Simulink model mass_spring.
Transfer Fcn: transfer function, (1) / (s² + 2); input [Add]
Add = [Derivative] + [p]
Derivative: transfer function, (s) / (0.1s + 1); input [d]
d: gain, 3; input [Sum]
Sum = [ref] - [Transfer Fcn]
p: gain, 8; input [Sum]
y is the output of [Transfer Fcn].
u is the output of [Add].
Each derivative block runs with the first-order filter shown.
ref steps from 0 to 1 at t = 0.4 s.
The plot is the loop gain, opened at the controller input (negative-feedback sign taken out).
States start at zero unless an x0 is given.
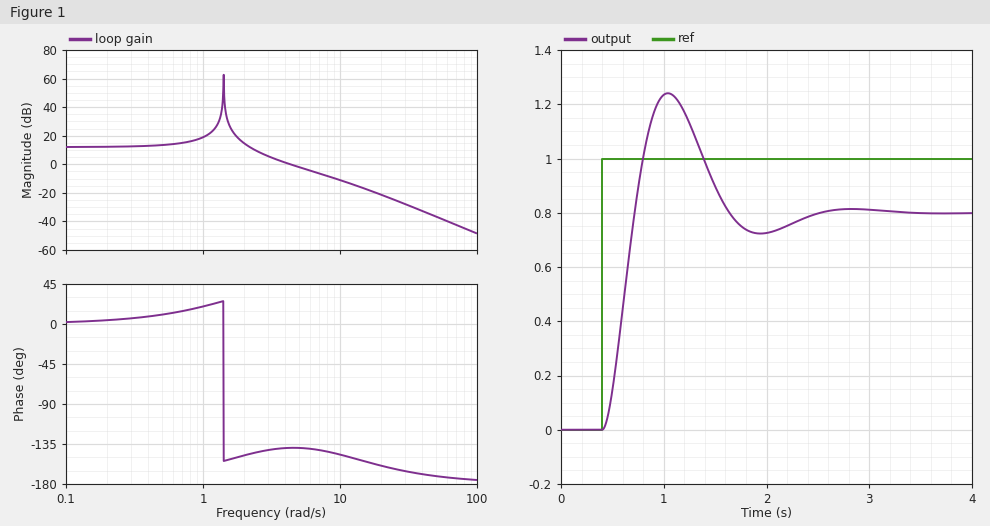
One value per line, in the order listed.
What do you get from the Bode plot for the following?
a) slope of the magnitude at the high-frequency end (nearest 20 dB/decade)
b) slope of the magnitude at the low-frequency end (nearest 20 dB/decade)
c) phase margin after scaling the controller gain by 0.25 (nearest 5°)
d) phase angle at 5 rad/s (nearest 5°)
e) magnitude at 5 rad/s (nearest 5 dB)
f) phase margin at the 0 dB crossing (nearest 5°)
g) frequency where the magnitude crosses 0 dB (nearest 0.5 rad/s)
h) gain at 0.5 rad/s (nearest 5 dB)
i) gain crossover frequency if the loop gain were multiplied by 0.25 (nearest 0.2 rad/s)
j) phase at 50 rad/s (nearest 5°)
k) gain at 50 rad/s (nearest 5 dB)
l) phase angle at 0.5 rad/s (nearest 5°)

-40 dB/decade
0 dB/decade
35°
-140°
0 dB
40°
4.5 rad/s
15 dB
2.2 rad/s
-170°
-35 dB
10°
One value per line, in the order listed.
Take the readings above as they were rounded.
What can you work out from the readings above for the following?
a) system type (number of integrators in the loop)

0
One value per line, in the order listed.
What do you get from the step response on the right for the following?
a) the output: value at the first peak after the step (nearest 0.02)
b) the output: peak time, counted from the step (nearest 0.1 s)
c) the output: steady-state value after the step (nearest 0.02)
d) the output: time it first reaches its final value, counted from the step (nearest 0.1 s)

1.24
0.6 s
0.80
0.3 s
